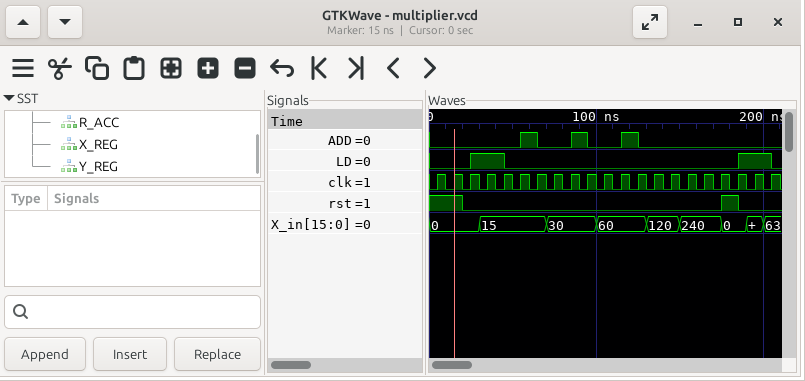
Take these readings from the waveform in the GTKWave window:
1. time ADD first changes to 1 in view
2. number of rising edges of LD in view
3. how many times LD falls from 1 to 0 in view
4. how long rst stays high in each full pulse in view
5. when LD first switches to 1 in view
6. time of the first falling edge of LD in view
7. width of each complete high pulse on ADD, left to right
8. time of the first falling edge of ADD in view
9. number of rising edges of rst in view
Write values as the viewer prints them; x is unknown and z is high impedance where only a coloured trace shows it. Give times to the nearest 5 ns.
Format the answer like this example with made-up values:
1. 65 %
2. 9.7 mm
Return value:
1. 55 ns
2. 2
3. 2
4. 10 ns
5. 25 ns
6. 45 ns
7. 10 ns, 10 ns, 10 ns
8. 65 ns
9. 1
